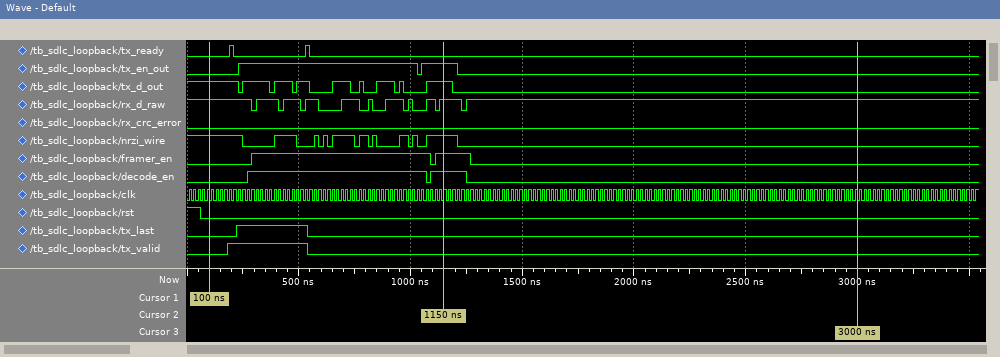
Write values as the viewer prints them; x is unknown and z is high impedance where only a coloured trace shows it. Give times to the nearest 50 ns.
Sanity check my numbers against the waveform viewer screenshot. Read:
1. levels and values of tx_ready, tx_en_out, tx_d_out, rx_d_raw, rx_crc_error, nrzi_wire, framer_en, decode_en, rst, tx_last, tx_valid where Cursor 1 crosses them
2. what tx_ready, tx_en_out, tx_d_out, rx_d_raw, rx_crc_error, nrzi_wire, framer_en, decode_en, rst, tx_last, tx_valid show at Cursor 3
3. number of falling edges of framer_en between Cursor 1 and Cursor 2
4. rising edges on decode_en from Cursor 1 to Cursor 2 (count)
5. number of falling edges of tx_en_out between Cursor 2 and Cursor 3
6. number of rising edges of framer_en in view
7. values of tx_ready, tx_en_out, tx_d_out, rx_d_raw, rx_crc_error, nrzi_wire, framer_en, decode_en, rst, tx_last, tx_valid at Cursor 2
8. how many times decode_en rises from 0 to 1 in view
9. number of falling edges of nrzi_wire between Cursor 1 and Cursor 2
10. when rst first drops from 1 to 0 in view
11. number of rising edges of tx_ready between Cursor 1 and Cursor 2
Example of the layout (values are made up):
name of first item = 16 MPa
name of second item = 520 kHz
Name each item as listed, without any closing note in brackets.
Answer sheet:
levels and values of tx_ready, tx_en_out, tx_d_out, rx_d_raw, rx_crc_error, nrzi_wire, framer_en, decode_en, rst, tx_last, tx_valid where Cursor 1 crosses them = tx_ready=0, tx_en_out=0, tx_d_out=1, rx_d_raw=1, rx_crc_error=0, nrzi_wire=1, framer_en=0, decode_en=0, rst=0, tx_last=0, tx_valid=0
what tx_ready, tx_en_out, tx_d_out, rx_d_raw, rx_crc_error, nrzi_wire, framer_en, decode_en, rst, tx_last, tx_valid show at Cursor 3 = tx_ready=0, tx_en_out=0, tx_d_out=0, rx_d_raw=1, rx_crc_error=0, nrzi_wire=0, framer_en=0, decode_en=0, rst=0, tx_last=0, tx_valid=0
number of falling edges of framer_en between Cursor 1 and Cursor 2 = 1
rising edges on decode_en from Cursor 1 to Cursor 2 = 2
number of falling edges of tx_en_out between Cursor 2 and Cursor 3 = 1
number of rising edges of framer_en in view = 2
values of tx_ready, tx_en_out, tx_d_out, rx_d_raw, rx_crc_error, nrzi_wire, framer_en, decode_en, rst, tx_last, tx_valid at Cursor 2 = tx_ready=0, tx_en_out=1, tx_d_out=1, rx_d_raw=1, rx_crc_error=0, nrzi_wire=1, framer_en=1, decode_en=1, rst=0, tx_last=0, tx_valid=0
how many times decode_en rises from 0 to 1 in view = 2
number of falling edges of nrzi_wire between Cursor 1 and Cursor 2 = 9
when rst first drops from 1 to 0 in view = 50 ns
number of rising edges of tx_ready between Cursor 1 and Cursor 2 = 2
